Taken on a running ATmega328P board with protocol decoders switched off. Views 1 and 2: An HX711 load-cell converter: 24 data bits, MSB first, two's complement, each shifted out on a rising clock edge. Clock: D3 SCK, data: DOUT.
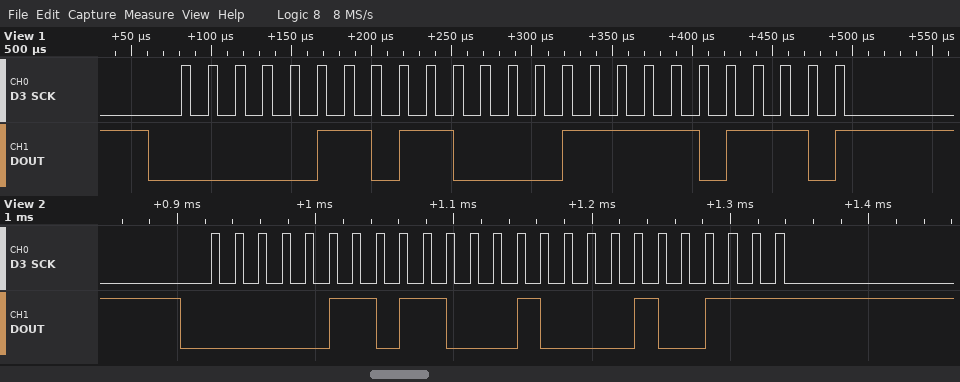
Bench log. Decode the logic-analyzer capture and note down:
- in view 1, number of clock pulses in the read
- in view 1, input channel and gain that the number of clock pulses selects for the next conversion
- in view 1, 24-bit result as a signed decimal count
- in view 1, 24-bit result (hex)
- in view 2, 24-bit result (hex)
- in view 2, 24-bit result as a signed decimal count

25
channel A, gain 128
443374
0x06C3EE
0x06C427
443431
